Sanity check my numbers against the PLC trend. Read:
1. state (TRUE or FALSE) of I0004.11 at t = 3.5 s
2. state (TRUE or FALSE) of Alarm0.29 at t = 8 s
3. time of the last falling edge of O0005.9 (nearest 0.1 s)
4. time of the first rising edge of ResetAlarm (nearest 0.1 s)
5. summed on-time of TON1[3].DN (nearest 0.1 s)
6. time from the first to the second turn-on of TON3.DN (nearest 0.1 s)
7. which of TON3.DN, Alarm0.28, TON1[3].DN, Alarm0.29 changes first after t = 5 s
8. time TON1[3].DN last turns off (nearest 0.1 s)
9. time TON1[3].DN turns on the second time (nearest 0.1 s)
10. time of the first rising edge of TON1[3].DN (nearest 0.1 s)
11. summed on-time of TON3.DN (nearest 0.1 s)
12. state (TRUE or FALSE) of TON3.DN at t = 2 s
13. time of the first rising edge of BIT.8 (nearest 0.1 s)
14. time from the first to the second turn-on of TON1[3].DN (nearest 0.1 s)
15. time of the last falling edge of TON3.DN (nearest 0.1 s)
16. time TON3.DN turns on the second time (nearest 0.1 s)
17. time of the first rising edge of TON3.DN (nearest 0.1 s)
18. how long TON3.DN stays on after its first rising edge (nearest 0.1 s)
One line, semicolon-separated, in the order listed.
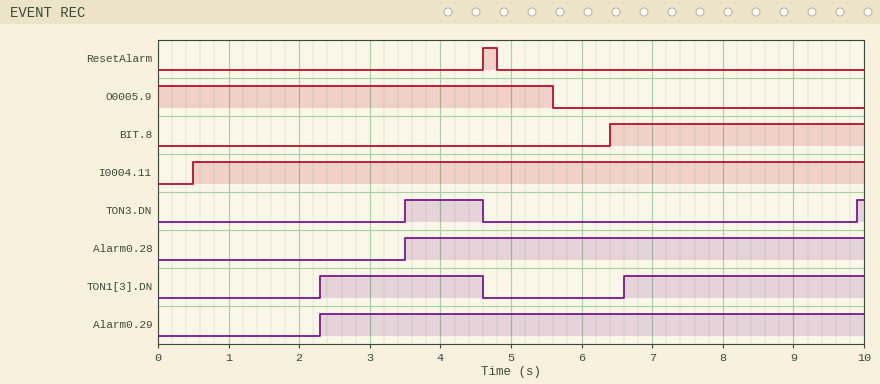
TRUE; TRUE; 5.6 s; 4.6 s; 5.7 s; 6.4 s; TON1[3].DN; 4.6 s; 6.6 s; 2.3 s; 1.2 s; FALSE; 6.4 s; 4.3 s; 4.6 s; 9.9 s; 3.5 s; 1.1 s
